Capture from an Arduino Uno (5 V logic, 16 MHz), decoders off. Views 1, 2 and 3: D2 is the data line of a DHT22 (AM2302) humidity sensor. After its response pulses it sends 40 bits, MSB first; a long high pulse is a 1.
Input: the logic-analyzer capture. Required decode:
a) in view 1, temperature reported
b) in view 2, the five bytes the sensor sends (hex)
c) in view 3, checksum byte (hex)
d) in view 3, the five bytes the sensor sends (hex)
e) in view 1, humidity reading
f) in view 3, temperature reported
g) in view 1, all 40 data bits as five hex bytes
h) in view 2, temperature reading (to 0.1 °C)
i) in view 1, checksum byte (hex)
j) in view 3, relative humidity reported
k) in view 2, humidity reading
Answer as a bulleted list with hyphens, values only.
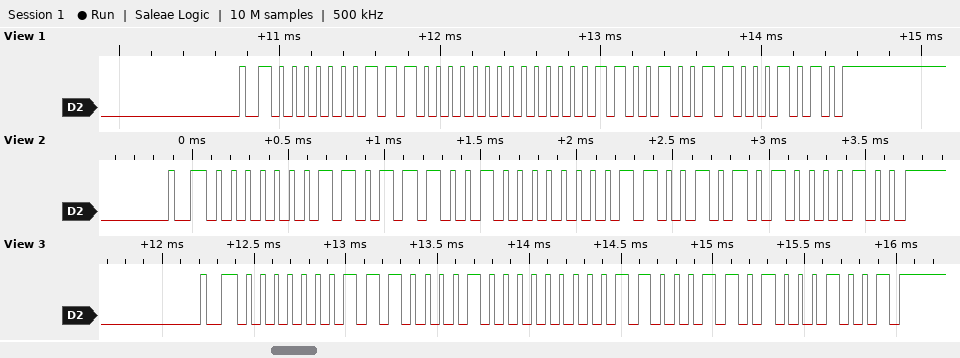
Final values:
- 20.1 °C
- 01 B9 00 CA 84
- 0x89
- 01 C2 00 C6 89
- 44.8 %
- 19.8 °C
- 01 C0 00 C9 8A
- 20.2 °C
- 0x8A
- 45.0 %
- 44.1 %
